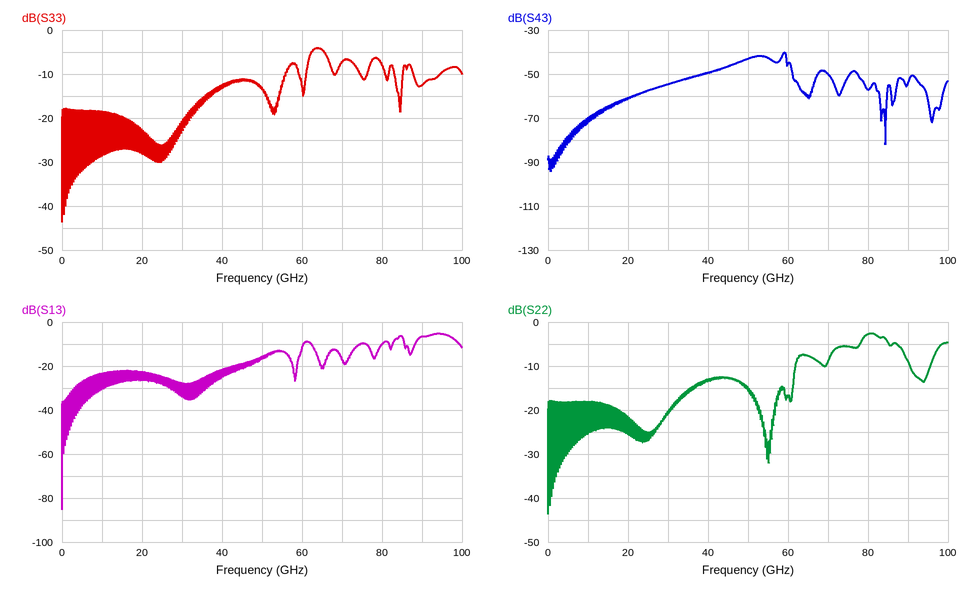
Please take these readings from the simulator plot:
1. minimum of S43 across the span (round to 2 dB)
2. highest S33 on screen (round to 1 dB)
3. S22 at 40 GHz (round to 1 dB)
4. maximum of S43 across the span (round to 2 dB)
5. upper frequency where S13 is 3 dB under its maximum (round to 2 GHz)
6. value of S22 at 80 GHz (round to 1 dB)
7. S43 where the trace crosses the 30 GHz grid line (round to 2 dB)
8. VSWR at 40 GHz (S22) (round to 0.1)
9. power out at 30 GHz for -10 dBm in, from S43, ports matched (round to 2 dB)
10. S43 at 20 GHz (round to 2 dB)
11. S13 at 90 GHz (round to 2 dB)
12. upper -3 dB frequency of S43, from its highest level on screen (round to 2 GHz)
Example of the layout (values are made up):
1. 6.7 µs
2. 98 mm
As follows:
1. -94 dB
2. -4 dB
3. -13 dB
4. -40 dB
5. 98 GHz
6. -3 dB
7. -54 dB
8. 1.6
9. -64 dBm
10. -60 dB
11. -6 dB
12. 60 GHz
